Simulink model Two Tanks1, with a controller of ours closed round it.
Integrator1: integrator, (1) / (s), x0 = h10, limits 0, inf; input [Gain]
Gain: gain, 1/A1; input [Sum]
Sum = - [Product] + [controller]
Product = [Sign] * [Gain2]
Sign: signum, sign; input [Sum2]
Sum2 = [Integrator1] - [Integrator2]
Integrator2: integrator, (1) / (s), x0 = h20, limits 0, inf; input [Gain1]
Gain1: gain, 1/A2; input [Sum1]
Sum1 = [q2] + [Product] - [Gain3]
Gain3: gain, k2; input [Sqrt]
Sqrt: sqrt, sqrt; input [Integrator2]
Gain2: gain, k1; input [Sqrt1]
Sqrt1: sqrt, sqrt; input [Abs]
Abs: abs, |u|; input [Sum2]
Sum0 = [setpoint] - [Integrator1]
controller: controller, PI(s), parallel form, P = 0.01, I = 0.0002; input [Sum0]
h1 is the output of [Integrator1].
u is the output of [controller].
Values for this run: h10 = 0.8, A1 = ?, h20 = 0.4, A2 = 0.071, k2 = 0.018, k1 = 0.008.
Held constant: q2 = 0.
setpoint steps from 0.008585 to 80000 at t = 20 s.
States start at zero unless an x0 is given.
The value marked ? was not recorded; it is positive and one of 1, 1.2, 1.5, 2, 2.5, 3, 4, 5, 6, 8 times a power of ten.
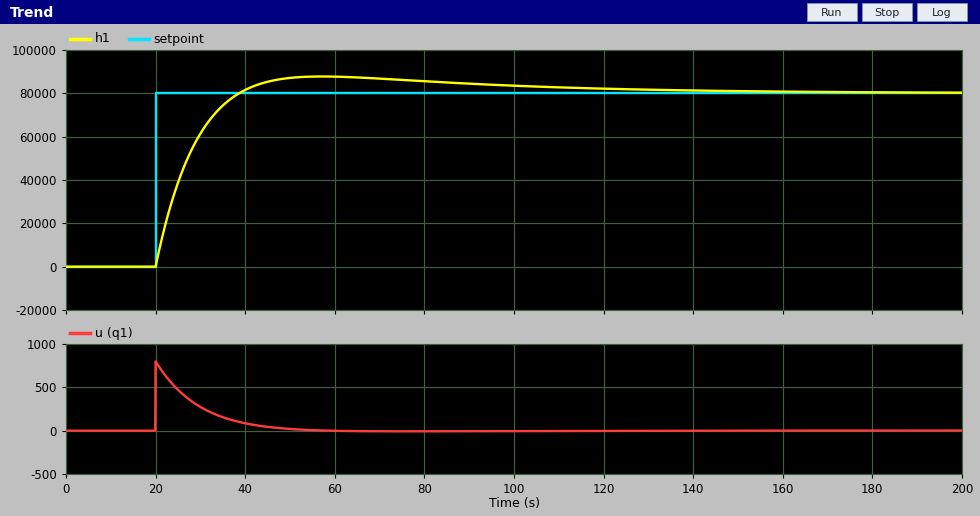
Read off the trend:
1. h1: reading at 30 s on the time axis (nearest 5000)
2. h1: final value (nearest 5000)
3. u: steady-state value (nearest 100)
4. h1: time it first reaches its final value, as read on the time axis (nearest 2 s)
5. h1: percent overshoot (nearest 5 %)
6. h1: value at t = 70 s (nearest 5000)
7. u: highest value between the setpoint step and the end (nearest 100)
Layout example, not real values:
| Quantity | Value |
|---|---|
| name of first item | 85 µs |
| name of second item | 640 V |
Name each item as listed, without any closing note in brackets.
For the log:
| Quantity | Value |
|---|---|
| h1: reading at 30 s on the time axis | 60000 |
| h1: final value | 80000 |
| u: steady-state value | 0 |
| h1: time it first reaches its final value, as read on the time axis | 38 s |
| h1: percent overshoot | 10 % |
| h1: value at t = 70 s | 85000 |
| u: highest value between the setpoint step and the end | 800 |
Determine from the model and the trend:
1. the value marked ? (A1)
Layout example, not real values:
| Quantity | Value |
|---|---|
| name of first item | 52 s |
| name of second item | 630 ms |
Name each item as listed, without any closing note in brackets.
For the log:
| Quantity | Value |
|---|---|
| the value marked ? | 0.08 |
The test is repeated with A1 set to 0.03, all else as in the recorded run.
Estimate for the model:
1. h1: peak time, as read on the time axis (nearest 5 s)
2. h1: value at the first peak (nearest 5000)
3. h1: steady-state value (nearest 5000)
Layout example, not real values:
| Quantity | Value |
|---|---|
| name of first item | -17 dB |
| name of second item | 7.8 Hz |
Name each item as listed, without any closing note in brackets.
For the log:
| Quantity | Value |
|---|---|
| h1: peak time, as read on the time axis | 40 s |
| h1: value at the first peak | 85000 |
| h1: steady-state value | 80000 |
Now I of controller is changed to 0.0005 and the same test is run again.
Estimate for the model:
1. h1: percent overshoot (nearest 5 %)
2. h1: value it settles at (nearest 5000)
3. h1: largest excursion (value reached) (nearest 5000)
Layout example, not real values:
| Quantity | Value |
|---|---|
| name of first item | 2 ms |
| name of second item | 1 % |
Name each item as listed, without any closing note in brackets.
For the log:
| Quantity | Value |
|---|---|
| h1: percent overshoot | 20 % |
| h1: value it settles at | 80000 |
| h1: largest excursion (value reached) | 95000 |
